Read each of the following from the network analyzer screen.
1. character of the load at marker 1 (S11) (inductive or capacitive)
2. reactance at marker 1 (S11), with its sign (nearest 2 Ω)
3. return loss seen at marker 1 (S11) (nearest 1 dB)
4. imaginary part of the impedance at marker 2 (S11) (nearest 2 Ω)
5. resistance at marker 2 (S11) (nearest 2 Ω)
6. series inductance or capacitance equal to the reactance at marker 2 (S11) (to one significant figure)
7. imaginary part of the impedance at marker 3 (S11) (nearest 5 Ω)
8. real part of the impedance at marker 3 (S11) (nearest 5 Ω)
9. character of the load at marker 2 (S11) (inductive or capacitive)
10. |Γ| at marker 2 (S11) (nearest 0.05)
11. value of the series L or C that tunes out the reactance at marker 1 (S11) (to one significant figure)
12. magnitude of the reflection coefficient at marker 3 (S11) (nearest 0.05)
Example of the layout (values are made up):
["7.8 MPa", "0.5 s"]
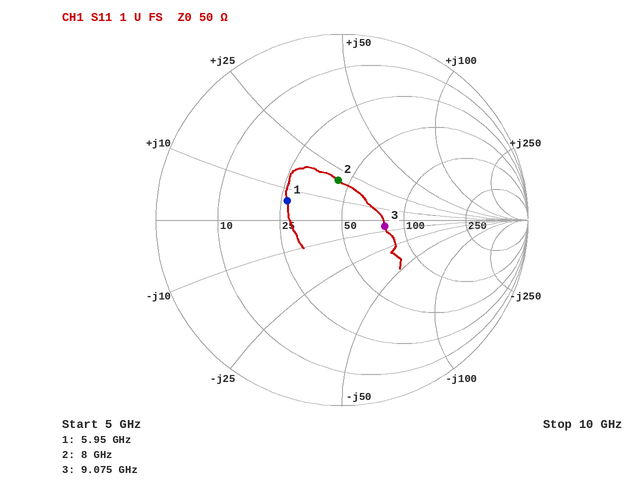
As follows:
["inductive", "+6 Ω", "10 dB", "+20 Ω", "44 Ω", "400 pH", "-5 Ω", "80 Ω", "inductive", "0.20", "4 pF", "0.25"]
